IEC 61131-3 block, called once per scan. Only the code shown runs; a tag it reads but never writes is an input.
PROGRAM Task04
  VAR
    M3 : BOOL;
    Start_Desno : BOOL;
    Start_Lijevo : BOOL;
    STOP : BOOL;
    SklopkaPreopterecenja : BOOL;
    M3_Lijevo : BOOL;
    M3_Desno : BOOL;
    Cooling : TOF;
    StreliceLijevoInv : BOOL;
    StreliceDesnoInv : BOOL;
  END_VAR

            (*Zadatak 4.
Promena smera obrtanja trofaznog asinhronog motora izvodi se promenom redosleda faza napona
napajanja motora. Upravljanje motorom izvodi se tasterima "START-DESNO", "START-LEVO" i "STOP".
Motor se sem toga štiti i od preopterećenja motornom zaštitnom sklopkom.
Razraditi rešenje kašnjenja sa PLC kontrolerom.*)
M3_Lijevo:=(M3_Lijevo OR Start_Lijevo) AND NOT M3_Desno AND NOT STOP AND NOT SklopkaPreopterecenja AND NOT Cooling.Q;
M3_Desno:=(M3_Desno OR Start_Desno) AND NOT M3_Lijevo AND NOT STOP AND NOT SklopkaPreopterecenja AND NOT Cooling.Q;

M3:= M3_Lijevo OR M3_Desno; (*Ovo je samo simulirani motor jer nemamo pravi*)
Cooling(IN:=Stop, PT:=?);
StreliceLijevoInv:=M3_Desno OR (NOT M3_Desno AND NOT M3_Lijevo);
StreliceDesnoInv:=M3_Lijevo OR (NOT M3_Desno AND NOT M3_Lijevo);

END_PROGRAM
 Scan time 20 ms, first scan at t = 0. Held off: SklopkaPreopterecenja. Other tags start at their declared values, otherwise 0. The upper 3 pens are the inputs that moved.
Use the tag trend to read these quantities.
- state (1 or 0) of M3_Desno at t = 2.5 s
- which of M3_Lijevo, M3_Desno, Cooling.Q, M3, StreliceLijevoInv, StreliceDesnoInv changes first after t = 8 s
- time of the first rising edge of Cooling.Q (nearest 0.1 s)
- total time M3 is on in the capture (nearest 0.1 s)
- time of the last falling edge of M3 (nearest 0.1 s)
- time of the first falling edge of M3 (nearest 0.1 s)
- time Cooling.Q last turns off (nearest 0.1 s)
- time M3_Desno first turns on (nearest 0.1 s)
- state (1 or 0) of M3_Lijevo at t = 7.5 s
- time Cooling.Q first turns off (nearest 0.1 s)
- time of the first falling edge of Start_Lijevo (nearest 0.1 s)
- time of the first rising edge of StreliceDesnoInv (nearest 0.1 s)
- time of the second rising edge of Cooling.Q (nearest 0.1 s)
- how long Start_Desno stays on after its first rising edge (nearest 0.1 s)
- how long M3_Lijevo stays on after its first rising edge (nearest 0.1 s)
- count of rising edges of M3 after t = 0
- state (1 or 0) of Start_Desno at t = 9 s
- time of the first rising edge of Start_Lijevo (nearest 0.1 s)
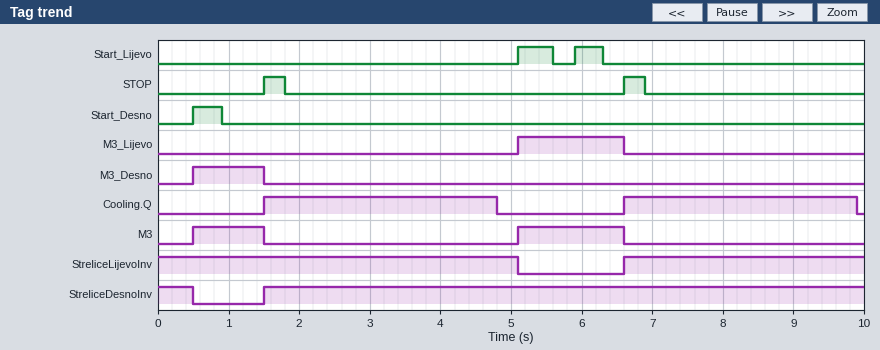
0
Cooling.Q
1.5 s
2.5 s
6.6 s
1.5 s
9.9 s
0.5 s
0
4.8 s
5.6 s
1.5 s
6.6 s
0.4 s
1.5 s
2
0
5.1 s
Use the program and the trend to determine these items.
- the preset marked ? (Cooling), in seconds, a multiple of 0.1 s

3.0 s
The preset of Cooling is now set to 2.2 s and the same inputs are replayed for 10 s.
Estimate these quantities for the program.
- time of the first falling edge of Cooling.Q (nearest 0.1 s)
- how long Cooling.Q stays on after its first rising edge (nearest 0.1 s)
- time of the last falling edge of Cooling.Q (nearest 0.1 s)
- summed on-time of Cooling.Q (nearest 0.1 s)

4.0 s
2.5 s
9.1 s
5.0 s
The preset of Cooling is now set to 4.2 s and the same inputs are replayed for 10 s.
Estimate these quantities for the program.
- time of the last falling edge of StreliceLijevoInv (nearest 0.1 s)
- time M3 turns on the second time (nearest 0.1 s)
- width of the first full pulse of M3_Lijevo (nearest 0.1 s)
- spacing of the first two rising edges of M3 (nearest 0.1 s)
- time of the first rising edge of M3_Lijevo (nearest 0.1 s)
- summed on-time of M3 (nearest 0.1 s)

6.0 s
6.0 s
0.6 s
5.5 s
6.0 s
1.6 s
